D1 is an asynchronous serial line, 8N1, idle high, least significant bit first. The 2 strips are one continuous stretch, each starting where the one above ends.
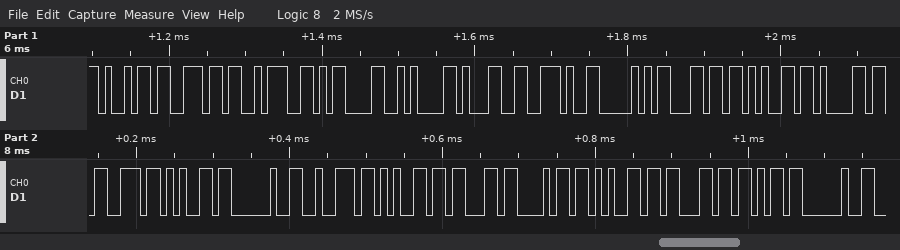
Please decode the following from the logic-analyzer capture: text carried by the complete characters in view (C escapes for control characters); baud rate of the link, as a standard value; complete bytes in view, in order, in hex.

"in:\r\n1.Please recheck "
115200 baud
0x69 0x6E 0x3A 0x0D 0x0A 0x31 0x2E 0x50 0x6C 0x65 0x61 0x73 0x65 0x20 0x72 0x65 0x63 0x68 0x65 0x63 0x6B 0x20
